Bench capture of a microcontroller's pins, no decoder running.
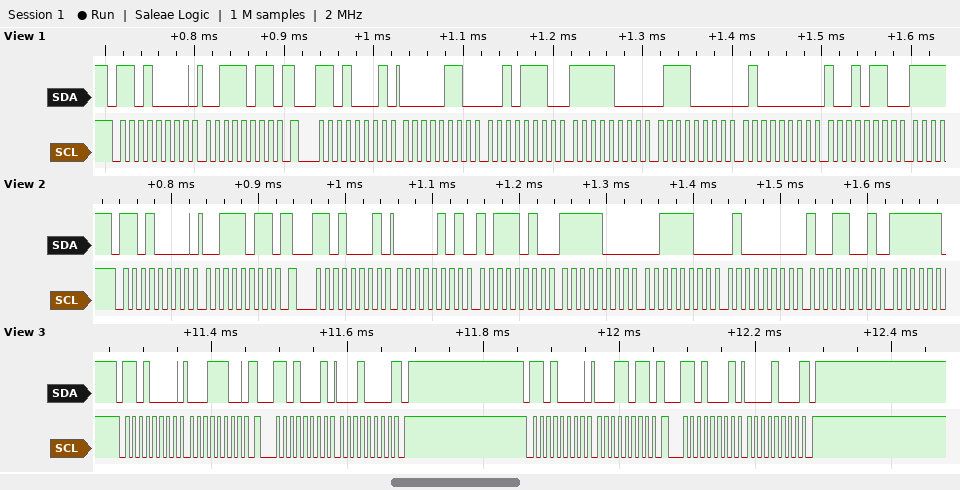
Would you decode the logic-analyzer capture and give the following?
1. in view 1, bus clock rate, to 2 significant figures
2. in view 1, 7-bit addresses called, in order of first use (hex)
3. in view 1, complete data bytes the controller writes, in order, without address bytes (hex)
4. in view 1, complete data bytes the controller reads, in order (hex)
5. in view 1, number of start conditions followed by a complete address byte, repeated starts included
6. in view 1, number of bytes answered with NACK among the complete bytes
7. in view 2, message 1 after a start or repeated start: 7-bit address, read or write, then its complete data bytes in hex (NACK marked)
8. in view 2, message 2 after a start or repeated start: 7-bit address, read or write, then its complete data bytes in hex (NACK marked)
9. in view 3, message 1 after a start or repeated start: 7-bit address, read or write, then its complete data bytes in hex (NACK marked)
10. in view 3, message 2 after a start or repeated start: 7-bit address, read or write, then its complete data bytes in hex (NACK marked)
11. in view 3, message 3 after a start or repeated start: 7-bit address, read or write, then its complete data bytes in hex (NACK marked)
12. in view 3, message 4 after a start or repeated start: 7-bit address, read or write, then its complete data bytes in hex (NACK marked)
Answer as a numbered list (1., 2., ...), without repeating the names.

1. 100 kHz
2. 0x68
3. 3B
4. 06 2E F8 70 40 96
5. 2
6. 0
7. 0x68 write: 3B
8. 0x68 read: 05 BA F8 3C 40 99
9. 0x68 write: 1C
10. 0x68 read: 10 NACK
11. 0x68 write: 1B
12. 0x68 read: 08 NACK
